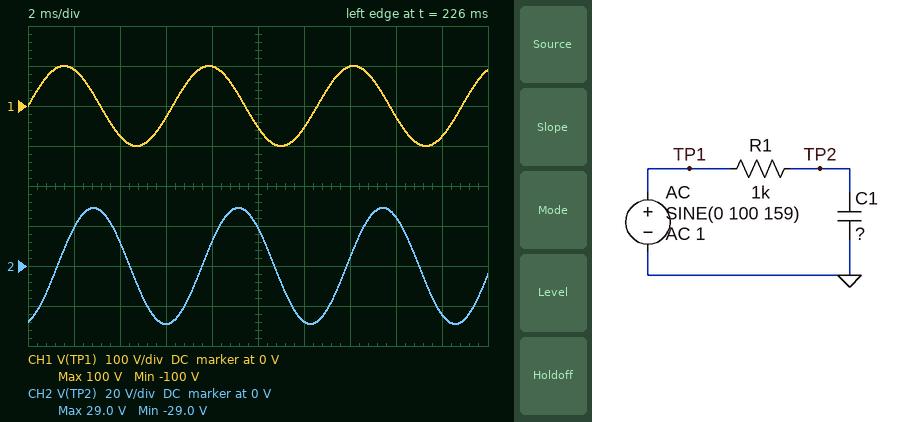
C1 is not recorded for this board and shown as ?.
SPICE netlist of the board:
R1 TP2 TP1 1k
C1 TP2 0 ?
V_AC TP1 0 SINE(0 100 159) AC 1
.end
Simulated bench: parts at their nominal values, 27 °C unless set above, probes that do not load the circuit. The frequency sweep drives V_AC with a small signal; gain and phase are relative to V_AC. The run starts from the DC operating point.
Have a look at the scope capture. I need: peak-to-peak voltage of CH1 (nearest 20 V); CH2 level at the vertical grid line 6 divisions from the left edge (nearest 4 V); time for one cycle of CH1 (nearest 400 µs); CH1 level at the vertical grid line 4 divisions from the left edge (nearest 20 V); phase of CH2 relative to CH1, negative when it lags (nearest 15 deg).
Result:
200 V
-28 V
6.4 ms
100 V
-75 deg
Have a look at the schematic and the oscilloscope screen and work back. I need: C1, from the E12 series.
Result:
3.3 µF
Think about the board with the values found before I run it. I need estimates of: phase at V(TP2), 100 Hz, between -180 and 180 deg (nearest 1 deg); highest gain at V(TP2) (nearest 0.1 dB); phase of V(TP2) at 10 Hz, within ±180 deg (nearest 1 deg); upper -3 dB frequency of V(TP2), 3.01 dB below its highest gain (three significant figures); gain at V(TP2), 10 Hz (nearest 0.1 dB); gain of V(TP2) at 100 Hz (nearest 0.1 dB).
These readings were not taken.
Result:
-64 deg
0 dB
-12 deg
48.2 Hz
-0.2 dB
-7.2 dB
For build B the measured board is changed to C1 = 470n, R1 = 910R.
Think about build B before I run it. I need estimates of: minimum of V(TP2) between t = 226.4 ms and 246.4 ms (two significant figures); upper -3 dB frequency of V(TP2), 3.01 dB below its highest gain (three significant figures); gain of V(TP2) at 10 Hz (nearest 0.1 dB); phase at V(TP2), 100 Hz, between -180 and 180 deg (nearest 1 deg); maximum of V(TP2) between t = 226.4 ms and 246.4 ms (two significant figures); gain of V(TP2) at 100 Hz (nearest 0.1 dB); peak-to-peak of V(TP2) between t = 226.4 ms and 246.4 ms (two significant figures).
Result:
-92 V
372 Hz
0 dB
-15 deg
92 V
-0.3 dB
180 V
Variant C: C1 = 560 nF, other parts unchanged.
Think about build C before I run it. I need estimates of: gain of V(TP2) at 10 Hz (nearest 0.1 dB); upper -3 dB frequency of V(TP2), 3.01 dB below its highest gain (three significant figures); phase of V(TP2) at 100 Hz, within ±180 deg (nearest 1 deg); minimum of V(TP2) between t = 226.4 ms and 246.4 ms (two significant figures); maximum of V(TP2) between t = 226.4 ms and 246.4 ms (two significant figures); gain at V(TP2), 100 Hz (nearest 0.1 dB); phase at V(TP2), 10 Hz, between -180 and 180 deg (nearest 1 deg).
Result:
0 dB
284 Hz
-19 deg
-87 V
87 V
-0.5 dB
-2 deg
